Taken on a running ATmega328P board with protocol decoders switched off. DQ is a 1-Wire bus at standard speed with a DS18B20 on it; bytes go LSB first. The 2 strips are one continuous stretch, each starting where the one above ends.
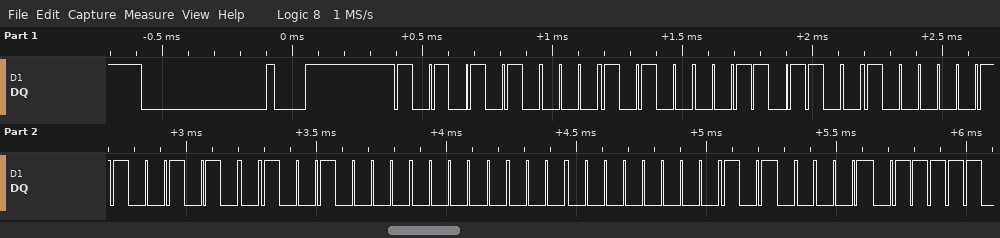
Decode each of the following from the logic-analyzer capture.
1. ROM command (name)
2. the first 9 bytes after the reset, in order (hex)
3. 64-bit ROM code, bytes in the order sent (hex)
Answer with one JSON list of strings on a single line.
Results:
["Match ROM", "55 28 6C 82 29 09 00 00 85", "28 6C 82 29 09 00 00 85"]
